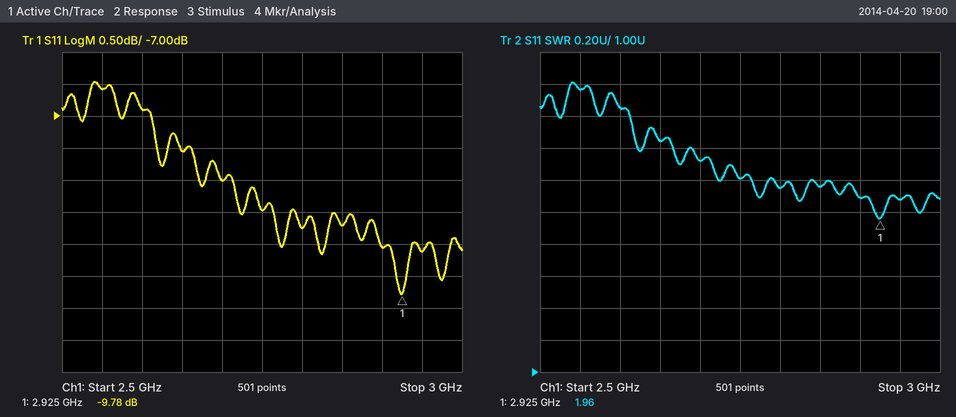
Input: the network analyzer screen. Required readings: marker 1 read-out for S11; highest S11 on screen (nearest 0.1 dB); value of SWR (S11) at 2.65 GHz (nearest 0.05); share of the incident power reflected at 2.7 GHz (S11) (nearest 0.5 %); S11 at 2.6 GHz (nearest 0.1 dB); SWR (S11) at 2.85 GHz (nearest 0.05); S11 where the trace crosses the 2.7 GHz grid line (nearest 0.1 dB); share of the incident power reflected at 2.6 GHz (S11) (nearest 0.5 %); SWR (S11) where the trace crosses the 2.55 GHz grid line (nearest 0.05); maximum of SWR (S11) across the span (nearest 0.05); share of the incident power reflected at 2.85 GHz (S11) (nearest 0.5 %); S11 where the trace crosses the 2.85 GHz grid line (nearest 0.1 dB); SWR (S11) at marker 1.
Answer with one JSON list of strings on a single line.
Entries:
["-9.78 dB", "-6.5 dB", "2.45", "16.0 %", "-6.9 dB", "2.15", "-8.0 dB", "20.5 %", "2.75", "2.80", "13.5 %", "-8.7 dB", "1.96"]
